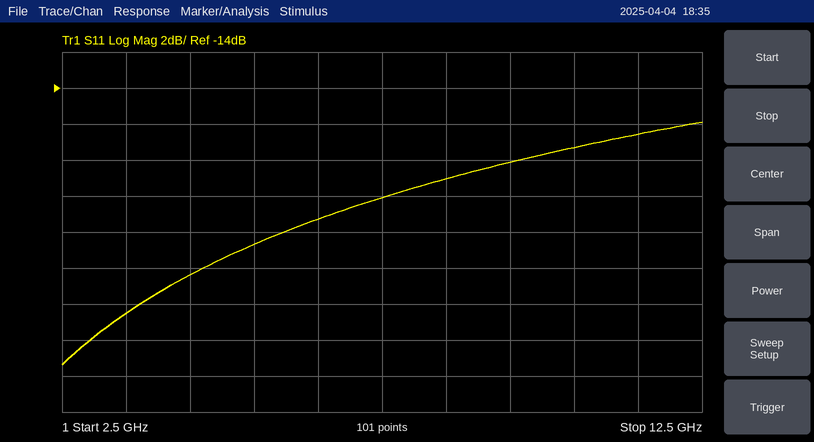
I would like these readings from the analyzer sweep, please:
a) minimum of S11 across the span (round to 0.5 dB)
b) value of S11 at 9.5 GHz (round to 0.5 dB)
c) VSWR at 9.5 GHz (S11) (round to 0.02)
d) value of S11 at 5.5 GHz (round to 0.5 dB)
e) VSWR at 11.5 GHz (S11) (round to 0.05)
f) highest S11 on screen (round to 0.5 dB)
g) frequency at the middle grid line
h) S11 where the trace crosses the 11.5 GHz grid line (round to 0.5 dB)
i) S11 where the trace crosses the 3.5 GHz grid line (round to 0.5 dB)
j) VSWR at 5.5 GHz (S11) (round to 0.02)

-29.5 dB
-18.0 dB
1.28
-22.5 dB
1.35
-16.0 dB
7.5 GHz
-16.5 dB
-26.5 dB
1.16
